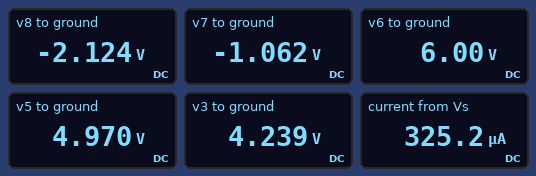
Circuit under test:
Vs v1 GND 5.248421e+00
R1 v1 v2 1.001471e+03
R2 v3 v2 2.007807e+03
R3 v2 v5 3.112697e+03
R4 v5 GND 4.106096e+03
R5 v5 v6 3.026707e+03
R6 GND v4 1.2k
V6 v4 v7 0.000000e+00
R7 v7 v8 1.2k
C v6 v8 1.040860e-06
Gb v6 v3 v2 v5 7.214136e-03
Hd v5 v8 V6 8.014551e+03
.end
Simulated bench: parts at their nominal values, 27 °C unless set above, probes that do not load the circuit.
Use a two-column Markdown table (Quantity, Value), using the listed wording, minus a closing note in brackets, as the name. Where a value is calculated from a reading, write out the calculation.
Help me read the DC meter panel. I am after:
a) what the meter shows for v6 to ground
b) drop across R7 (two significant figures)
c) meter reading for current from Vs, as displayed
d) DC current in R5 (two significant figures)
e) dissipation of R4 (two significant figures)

| Quantity | Value |
|---|---|
| what the meter shows for v6 to ground | 6.00 V |
| drop across R7 | -1.062 V - (-2.124 V) = 1.1 V |
| meter reading for current from Vs, as displayed | 325.2 µA |
| DC current in R5 | (6 V - 4.97 V) / 3.027 kΩ = 340 µA |
| dissipation of R4 | (4.97 V)^2 / 4.106 kΩ = 6.0 mW |
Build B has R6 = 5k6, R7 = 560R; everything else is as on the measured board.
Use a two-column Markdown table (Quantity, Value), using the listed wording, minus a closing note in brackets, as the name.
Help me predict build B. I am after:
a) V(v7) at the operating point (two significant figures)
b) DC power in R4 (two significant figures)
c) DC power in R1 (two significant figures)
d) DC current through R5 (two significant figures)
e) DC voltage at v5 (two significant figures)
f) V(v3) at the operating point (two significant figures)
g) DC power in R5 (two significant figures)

| Quantity | Value |
|---|---|
| V(v7) at the operating point | -21 V |
| DC power in R4 | 12 mW |
| DC power in R1 | 4.3 mW |
| DC current through R5 | 2.2 mA |
| DC voltage at v5 | 7.0 V |
| V(v3) at the operating point | 12 V |
| DC power in R5 | 14 mW |
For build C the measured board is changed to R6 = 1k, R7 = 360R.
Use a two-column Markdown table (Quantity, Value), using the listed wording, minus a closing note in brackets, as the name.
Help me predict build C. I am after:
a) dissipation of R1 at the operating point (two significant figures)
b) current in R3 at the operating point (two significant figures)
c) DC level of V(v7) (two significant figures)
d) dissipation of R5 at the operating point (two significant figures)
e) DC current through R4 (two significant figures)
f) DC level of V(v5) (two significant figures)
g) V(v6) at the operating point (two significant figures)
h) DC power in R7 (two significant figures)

| Quantity | Value |
|---|---|
| dissipation of R1 at the operating point | 210 µW |
| current in R3 at the operating point | 21 µA |
| DC level of V(v7) | -730 mV |
| dissipation of R5 at the operating point | 680 µW |
| DC current through R4 | 1.2 mA |
| DC level of V(v5) | 4.9 V |
| V(v6) at the operating point | 6.3 V |
| DC power in R7 | 190 µW |
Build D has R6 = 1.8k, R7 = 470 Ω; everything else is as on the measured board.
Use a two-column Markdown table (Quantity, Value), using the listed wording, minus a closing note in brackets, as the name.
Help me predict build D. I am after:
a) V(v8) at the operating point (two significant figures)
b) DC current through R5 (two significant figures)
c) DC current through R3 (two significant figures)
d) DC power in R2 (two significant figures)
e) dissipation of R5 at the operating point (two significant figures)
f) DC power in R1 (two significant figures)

| Quantity | Value |
|---|---|
| V(v8) at the operating point | -2.0 V |
| DC current through R5 | 360 µA |
| DC current through R3 | 16 µA |
| DC power in R2 | 260 µW |
| dissipation of R5 at the operating point | 390 µW |
| DC power in R1 | 120 µW |
